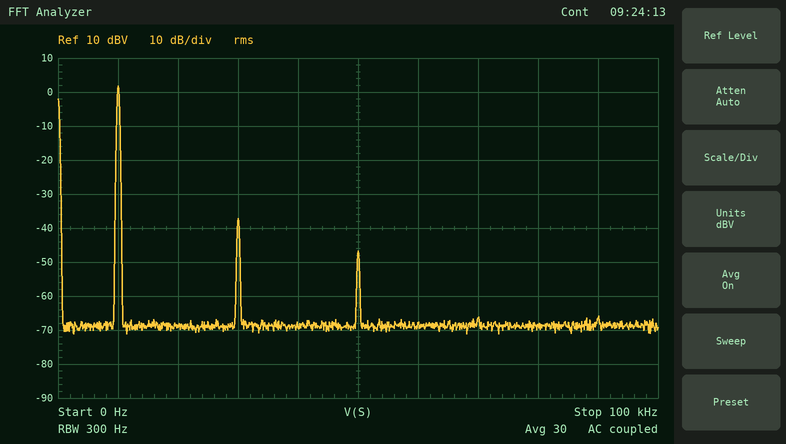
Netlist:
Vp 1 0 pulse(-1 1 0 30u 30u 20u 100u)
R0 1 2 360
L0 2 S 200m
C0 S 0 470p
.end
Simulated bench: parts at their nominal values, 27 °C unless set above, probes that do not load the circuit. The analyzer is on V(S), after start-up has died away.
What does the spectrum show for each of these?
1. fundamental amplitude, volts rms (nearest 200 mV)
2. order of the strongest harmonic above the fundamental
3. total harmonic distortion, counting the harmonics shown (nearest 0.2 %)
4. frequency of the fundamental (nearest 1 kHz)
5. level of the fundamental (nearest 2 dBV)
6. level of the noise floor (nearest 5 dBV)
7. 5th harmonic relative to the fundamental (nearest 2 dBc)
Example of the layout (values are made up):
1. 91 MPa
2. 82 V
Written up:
1. 1.2 V
2. 3
3. 1.2 %
4. 10 kHz
5. 2 dBV
6. -70 dBV
7. -48 dBc
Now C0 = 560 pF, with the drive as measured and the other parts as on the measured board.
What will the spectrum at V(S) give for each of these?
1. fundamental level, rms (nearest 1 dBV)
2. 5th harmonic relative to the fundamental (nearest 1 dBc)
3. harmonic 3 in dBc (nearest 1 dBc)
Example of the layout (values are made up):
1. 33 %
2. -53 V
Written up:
1. 3 dBV
2. -51 dBc
3. -42 dBc
